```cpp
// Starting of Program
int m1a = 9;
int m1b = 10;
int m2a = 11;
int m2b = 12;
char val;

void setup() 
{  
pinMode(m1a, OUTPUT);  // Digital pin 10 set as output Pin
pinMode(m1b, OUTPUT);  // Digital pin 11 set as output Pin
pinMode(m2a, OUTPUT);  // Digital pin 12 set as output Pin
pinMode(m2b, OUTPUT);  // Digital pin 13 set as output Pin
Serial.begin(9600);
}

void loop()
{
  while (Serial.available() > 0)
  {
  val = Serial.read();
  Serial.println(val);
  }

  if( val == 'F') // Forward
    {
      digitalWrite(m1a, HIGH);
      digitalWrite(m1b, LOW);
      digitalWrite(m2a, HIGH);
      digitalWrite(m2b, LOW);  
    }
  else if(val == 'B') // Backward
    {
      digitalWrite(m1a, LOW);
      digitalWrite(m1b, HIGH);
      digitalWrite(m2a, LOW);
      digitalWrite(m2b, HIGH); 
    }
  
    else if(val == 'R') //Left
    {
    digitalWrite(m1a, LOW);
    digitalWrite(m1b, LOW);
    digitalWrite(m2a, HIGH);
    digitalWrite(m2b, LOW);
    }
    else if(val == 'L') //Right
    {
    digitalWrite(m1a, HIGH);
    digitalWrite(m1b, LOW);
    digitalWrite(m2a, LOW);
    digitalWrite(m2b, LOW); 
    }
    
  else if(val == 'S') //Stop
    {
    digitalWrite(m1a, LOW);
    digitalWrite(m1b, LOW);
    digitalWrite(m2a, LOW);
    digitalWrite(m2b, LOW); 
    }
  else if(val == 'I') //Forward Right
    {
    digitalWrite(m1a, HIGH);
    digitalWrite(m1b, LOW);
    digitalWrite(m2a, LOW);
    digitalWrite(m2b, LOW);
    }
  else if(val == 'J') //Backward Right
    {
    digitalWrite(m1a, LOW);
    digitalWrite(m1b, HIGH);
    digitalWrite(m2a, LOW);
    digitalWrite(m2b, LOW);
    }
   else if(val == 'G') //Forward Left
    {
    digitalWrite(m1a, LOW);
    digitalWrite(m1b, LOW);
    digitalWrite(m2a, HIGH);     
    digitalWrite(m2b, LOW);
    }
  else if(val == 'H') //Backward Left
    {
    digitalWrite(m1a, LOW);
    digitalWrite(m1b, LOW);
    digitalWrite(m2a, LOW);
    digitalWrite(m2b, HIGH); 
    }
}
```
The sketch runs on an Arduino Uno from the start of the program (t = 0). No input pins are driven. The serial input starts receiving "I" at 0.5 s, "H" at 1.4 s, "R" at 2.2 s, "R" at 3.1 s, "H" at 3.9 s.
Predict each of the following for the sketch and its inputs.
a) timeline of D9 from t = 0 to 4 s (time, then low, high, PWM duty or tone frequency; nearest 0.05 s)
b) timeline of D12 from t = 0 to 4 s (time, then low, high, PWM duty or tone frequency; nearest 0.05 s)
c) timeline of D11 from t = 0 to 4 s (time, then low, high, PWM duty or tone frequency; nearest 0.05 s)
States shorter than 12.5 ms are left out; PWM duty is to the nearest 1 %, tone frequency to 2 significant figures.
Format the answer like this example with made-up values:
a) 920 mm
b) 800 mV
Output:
a) 0 s low; 0.5 s high; 1.4 s low
b) 0 s low; 1.4 s high; 2.2 s low; 3.9 s high
c) 0 s low; 2.2 s high; 3.9 s low
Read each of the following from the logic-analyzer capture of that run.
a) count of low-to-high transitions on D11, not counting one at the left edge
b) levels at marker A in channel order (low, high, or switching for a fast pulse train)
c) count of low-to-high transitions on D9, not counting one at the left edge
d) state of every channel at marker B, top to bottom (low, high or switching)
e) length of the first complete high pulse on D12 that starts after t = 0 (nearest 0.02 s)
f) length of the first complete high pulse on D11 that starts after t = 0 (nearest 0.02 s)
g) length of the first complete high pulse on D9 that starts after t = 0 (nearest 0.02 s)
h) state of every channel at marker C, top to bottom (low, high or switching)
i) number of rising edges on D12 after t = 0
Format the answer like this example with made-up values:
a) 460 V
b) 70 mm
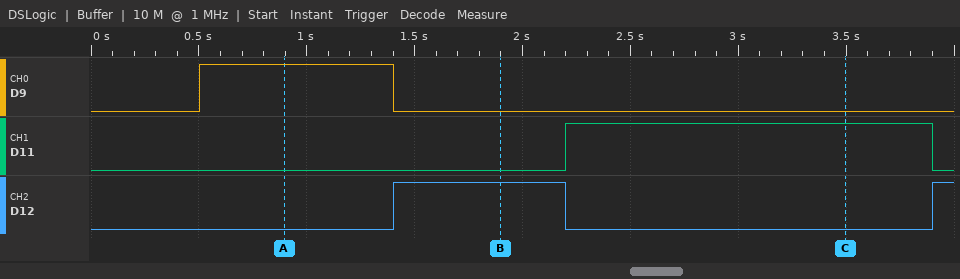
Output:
a) 1
b) D9 high, D11 low, D12 low
c) 1
d) D9 low, D11 low, D12 high
e) 0.80 s
f) 1.70 s
g) 0.90 s
h) D9 low, D11 high, D12 low
i) 2
